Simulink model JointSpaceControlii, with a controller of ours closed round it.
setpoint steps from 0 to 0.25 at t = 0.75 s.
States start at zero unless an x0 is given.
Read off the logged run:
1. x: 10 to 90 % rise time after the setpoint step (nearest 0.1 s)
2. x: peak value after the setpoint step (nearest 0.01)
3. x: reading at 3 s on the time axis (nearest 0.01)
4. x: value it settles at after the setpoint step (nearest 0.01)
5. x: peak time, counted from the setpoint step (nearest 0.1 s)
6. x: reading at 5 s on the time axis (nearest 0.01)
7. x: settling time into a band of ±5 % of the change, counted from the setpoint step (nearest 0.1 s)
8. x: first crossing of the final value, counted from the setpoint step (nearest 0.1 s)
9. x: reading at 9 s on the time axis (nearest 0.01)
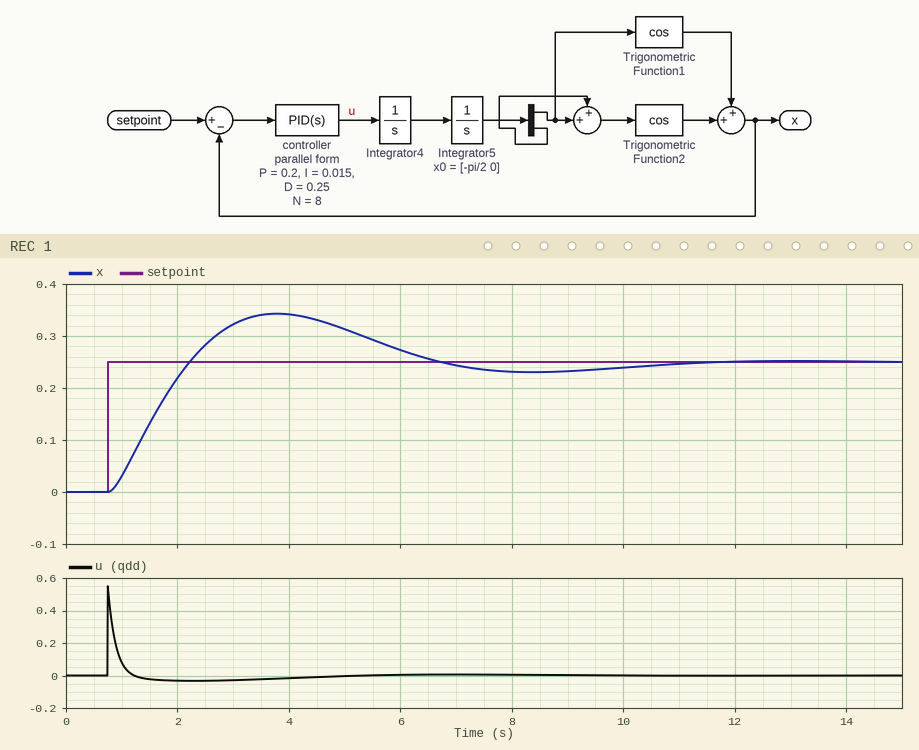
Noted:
1.1 s
0.34
0.32
0.25
3.0 s
0.31
9.0 s
1.5 s
0.23
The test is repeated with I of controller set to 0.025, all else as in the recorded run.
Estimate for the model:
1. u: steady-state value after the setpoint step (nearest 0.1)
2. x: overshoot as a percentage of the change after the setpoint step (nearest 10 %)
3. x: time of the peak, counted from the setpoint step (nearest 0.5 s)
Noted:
0.0
40 %
3.0 s
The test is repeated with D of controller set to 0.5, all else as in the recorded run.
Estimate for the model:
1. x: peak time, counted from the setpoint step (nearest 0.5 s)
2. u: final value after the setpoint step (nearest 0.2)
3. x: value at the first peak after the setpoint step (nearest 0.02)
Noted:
2.5 s
0.0
0.30
